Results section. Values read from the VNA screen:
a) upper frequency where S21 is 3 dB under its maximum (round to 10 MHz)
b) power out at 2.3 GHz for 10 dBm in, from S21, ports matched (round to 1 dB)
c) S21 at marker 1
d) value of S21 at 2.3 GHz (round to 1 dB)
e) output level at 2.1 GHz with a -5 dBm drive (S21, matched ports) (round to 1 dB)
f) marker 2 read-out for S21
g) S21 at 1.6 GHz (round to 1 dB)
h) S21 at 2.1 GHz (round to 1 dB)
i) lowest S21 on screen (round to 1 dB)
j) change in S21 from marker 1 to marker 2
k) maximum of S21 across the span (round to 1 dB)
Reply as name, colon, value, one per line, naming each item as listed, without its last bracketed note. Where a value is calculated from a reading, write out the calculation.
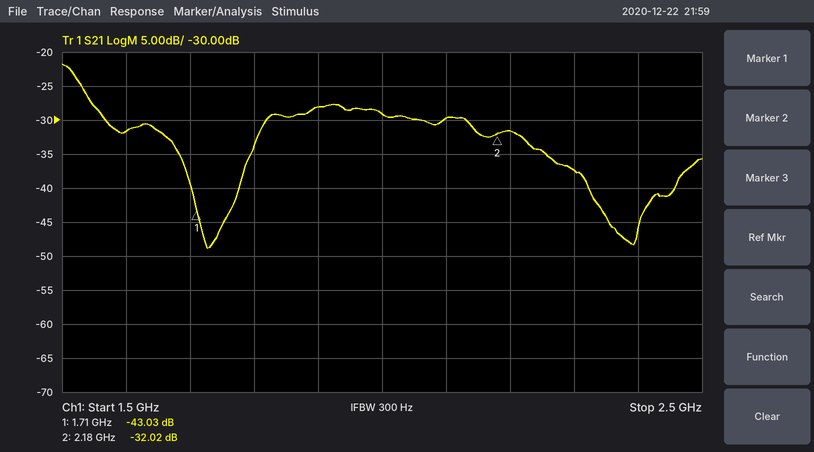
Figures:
upper frequency where S21 is 3 dB under its maximum: 1.53 GHz
power out at 2.3 GHz for 10 dBm in, from S21, ports matched: 10 dBm + (-37 dB) = -27 dBm
S21 at marker 1: -43.03 dB
value of S21 at 2.3 GHz: -37 dB
output level at 2.1 GHz with a -5 dBm drive (S21, matched ports): -5 dBm + (-30 dB) = -35 dBm
marker 2 read-out for S21: -32.02 dB
S21 at 1.6 GHz: -32 dB
S21 at 2.1 GHz: -30 dB
lowest S21 on screen: -49 dB
change in S21 from marker 1 to marker 2: -32.02 − (-43.03) = 11.01 dB
maximum of S21 across the span: -22 dB
